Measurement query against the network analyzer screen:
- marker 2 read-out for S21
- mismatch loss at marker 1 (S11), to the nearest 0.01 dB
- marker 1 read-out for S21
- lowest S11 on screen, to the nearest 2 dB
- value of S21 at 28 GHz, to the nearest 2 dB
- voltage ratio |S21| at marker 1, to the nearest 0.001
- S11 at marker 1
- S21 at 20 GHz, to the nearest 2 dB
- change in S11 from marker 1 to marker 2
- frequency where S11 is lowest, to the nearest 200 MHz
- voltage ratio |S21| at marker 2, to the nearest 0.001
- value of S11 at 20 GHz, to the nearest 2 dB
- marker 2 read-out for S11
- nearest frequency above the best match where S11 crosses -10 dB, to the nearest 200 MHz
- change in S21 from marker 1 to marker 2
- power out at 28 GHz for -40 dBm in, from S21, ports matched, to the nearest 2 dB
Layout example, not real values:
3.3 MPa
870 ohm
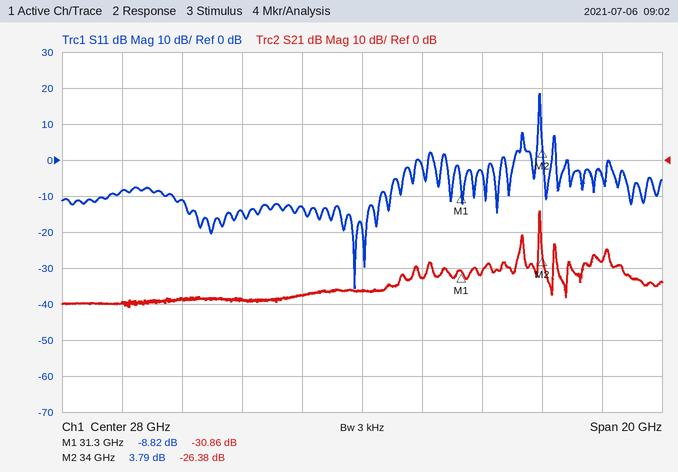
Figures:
-26.38 dB
0.61 dB
-30.86 dB
-36 dB
-36 dB
0.029
-8.82 dB
-40 dB
12.61 dB
27.8 GHz
0.048
-8 dB
3.79 dB
28.6 GHz
4.48 dB
-76 dBm
